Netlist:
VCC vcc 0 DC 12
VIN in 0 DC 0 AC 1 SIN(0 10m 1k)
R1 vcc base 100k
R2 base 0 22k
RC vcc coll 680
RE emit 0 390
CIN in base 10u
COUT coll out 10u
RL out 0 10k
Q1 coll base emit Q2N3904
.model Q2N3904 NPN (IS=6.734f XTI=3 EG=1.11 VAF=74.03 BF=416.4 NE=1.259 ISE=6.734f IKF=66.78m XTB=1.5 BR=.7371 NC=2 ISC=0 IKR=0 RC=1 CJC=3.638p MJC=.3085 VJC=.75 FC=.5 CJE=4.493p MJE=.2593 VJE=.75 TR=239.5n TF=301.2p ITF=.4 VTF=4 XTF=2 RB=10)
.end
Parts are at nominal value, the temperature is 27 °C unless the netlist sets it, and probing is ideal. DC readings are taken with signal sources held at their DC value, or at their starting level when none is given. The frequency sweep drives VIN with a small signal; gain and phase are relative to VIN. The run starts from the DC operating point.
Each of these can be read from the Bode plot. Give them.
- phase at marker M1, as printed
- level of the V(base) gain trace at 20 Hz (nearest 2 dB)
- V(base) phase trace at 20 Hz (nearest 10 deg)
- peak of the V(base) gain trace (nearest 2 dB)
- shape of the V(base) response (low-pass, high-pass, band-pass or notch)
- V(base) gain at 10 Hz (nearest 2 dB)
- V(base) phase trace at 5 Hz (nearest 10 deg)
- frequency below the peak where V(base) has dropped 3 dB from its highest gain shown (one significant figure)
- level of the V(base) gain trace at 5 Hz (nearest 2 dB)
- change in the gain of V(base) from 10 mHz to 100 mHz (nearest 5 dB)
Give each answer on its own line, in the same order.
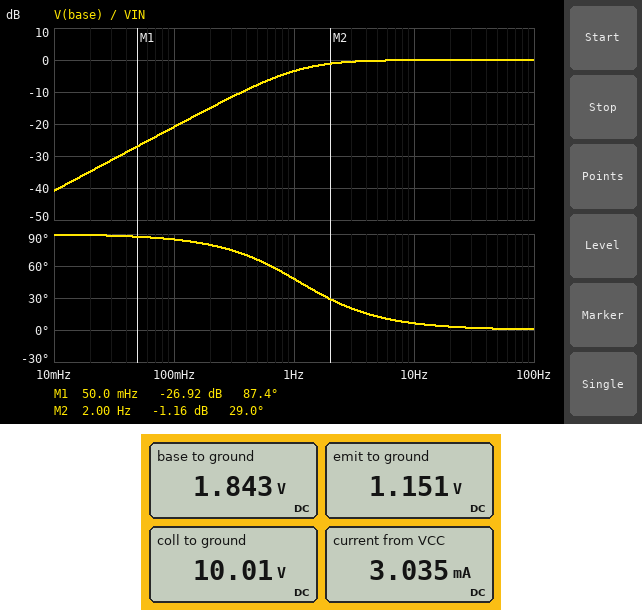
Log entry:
87.4 deg
0 dB
0 deg
0 dB
high-pass
0 dB
10 deg
1 Hz
0 dB
20 dB
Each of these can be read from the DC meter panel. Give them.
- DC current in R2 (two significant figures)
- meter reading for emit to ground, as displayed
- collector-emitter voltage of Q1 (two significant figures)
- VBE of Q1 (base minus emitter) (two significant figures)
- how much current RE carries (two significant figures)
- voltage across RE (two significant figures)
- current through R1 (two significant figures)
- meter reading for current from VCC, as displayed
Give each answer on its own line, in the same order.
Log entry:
84 µA
1.151 V
8.9 V
690 mV
3.0 mA
1.2 V
100 µA
3.035 mA
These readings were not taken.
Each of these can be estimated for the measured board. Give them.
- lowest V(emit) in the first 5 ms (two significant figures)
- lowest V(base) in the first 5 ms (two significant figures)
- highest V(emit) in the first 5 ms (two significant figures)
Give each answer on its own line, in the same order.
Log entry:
1.1 V
1.8 V
1.2 V
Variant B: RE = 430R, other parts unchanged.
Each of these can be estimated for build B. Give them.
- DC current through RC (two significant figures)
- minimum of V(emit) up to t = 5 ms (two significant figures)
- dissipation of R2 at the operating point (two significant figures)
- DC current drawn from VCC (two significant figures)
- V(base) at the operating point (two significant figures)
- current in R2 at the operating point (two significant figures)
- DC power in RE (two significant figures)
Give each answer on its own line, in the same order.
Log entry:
2.7 mA
1.2 V
160 µW
2.8 mA
1.9 V
85 µA
3.2 mW
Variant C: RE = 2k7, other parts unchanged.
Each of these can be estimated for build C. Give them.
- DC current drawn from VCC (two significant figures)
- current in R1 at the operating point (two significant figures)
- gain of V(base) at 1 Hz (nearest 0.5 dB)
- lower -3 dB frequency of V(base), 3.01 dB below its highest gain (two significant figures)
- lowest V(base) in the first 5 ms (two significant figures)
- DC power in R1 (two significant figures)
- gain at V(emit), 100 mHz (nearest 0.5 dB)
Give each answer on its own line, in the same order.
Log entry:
630 µA
99 µA
-2.5 dB
920 mHz
2.1 V
980 µW
-19.5 dB
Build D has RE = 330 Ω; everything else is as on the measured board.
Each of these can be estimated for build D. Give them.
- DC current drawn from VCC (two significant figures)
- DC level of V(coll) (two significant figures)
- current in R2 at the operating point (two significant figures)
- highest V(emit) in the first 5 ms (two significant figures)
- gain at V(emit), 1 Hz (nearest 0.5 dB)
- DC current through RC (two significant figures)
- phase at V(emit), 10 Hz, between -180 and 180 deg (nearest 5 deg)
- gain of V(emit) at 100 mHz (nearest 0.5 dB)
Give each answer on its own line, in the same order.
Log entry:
3.4 mA
9.7 V
82 µA
1.1 V
-4.0 dB
3.3 mA
5 deg
-21.5 dB
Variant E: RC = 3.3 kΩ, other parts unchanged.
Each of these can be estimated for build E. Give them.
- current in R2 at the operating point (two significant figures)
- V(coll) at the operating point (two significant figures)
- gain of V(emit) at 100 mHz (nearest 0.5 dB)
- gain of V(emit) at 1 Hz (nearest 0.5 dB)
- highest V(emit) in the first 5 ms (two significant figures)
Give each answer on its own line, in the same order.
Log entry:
83 µA
2.5 V
-21.5 dB
-4.0 dB
1.1 V
